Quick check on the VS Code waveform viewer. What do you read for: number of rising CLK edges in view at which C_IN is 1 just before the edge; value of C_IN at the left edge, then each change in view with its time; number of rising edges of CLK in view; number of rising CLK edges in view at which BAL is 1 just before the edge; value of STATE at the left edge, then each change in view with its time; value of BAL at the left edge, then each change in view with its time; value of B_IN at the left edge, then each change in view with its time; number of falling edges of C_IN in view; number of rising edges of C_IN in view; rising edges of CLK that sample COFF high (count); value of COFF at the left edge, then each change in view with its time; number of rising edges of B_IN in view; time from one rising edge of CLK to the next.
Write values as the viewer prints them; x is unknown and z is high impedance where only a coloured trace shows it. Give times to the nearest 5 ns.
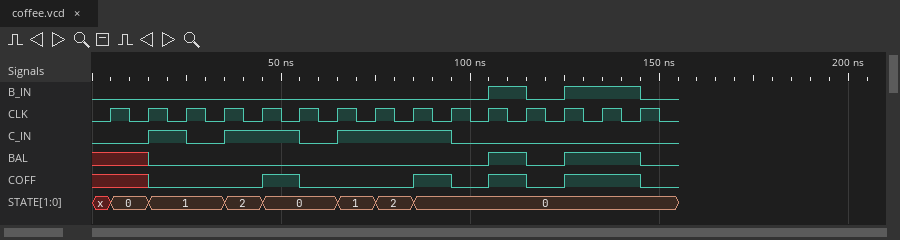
6
0, 1 at 15 ns, 0 at 25 ns, 1 at 35 ns, 0 at 55 ns, 1 at 65 ns, 0 at 95 ns
15
3
x, 0 at 5 ns, 1 at 15 ns, 2 at 35 ns, 0 at 45 ns, 1 at 65 ns, 2 at 75 ns, 0 at 85 ns
x, 0 at 15 ns, 1 at 105 ns, 0 at 115 ns, 1 at 125 ns, 0 at 145 ns
0, 1 at 105 ns, 0 at 115 ns, 1 at 125 ns, 0 at 145 ns
3
3
5
x, 0 at 15 ns, 1 at 45 ns, 0 at 55 ns, 1 at 85 ns, 0 at 95 ns, 1 at 105 ns, 0 at 115 ns, 1 at 125 ns, 0 at 145 ns
2
10 ns
